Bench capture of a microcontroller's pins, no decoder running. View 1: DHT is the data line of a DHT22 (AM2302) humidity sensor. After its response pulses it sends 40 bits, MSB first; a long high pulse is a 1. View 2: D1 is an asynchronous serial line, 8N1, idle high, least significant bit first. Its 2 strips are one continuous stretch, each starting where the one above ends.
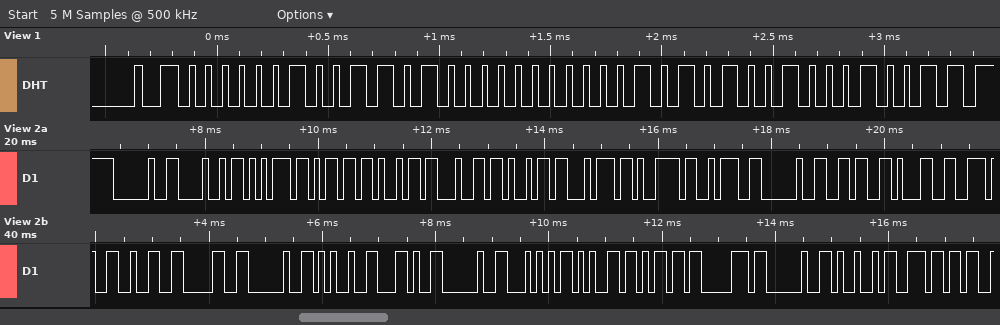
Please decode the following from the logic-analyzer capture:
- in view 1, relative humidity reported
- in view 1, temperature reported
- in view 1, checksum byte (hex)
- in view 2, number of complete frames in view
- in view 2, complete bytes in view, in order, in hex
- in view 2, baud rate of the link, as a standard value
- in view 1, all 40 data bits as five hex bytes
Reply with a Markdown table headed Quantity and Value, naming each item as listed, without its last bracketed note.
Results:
| Quantity | Value |
|---|---|
| in view 1, relative humidity reported | 61.6 % |
| in view 1, temperature reported | 16.9 °C |
| in view 1, checksum byte | 0x13 |
| in view 2, number of complete frames in view | 27 |
| in view 2, complete bytes in view, in order, in hex | 0x20 0x48 0x75 0x6D 0x69 0x64 0x69 0x74 0x79 0x3A 0x20 0x36 0x31 0x2E 0x32 0x30 0x20 0x25 0x2C 0x20 0x54 0x65 0x6D 0x70 0x20 0x49 0x6E |
| in view 2, baud rate of the link, as a standard value | 9600 baud |
| in view 1, all 40 data bits as five hex bytes | 02 68 00 A9 13 |
